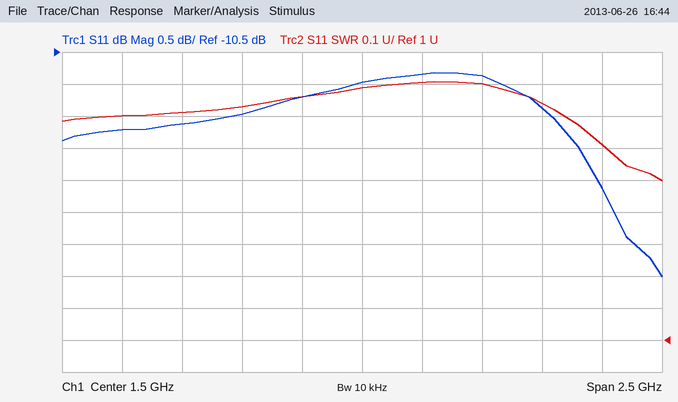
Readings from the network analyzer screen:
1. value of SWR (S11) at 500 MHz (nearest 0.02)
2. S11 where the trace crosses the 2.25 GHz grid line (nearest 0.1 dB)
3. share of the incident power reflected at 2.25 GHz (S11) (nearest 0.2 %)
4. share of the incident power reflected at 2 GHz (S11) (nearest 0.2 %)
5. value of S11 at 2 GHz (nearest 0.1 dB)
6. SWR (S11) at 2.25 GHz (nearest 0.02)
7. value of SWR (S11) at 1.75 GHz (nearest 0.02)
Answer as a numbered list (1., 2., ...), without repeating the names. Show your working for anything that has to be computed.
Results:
1. 1.70
2. -11.4 dB
3. 10^(-11.4/10) ≈ 7.2 %
4. 10^(-10.9/10) ≈ 8.13 %, so 8.2 % to the nearest 0.2 %
5. -10.9 dB
6. 1.74
7. 1.80
